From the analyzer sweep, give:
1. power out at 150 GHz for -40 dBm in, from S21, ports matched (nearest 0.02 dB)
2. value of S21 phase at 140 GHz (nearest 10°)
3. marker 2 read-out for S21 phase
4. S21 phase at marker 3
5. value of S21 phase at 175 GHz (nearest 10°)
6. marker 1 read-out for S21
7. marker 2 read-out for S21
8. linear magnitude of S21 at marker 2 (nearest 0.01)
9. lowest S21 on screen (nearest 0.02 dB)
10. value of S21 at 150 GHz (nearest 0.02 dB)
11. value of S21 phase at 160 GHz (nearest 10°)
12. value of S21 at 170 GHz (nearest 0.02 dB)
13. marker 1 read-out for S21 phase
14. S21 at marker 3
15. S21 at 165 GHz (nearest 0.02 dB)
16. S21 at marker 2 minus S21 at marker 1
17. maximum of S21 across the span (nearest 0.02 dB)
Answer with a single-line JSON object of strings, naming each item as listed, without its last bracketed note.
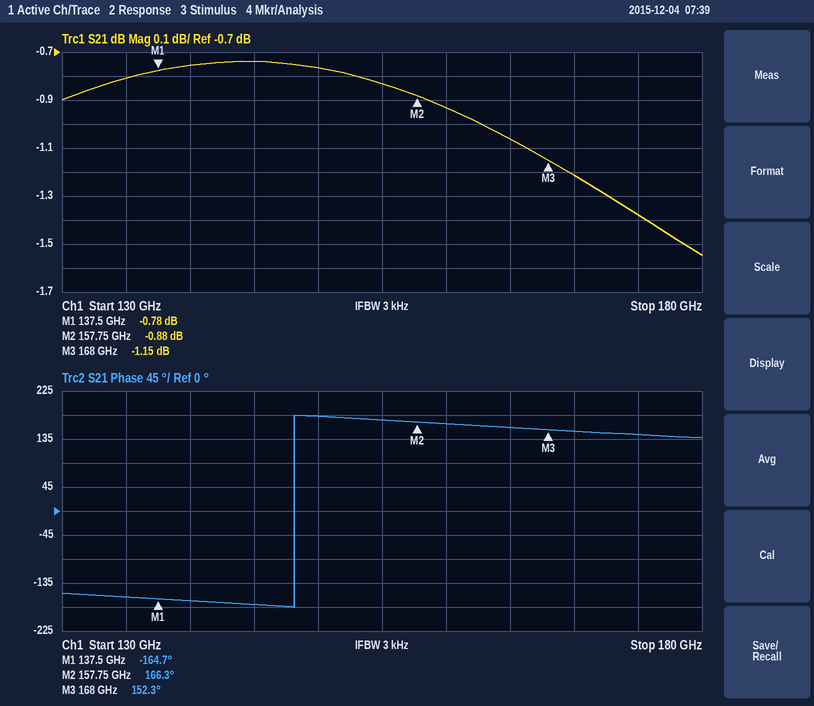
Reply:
{"power out at 150 GHz for -40 dBm in, from S21, ports matched": "-40.76 dBm", "value of S21 phase at 140 GHz": "-170°", "marker 2 read-out for S21 phase": "166.3°", "S21 phase at marker 3": "152.3°", "value of S21 phase at 175 GHz": "140°", "marker 1 read-out for S21": "-0.78 dB", "marker 2 read-out for S21": "-0.88 dB", "linear magnitude of S21 at marker 2": "0.90", "lowest S21 on screen": "-1.54 dB", "value of S21 at 150 GHz": "-0.76 dB", "value of S21 phase at 160 GHz": "160°", "value of S21 at 170 GHz": "-1.22 dB", "marker 1 read-out for S21 phase": "-164.7°", "S21 at marker 3": "-1.15 dB", "S21 at 165 GHz": "-1.06 dB", "S21 at marker 2 minus S21 at marker 1": "-0.10 dB", "maximum of S21 across the span": "-0.74 dB"}
